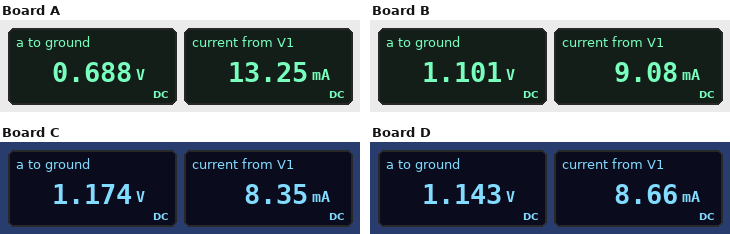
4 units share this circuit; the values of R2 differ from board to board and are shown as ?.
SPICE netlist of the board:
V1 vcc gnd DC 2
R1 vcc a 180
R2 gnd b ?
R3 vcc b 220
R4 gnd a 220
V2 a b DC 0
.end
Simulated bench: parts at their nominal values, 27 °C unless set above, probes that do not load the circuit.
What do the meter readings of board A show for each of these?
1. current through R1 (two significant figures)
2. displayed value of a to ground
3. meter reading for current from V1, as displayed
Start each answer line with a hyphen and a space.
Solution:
- 7.3 mA
- 0.688 V
- 13.25 mA
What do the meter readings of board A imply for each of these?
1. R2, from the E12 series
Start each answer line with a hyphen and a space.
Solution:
- 68 Ω
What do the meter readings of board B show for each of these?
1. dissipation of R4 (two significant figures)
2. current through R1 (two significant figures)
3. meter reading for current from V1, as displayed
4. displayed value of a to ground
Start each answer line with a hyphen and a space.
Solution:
- 5.5 mW
- 5.0 mA
- 9.08 mA
- 1.101 V
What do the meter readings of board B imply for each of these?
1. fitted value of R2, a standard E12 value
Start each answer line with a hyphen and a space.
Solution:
- 270 Ω
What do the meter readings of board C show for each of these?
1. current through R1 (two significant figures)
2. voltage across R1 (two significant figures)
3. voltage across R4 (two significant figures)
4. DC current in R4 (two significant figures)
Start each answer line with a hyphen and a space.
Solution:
- 4.6 mA
- 830 mV
- 1.2 V
- 5.3 mA
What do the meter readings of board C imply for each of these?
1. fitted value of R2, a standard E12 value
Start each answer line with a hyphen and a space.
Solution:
- 390 Ω
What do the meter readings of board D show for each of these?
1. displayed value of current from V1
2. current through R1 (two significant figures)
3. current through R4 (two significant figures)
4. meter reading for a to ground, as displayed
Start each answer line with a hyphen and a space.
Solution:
- 8.66 mA
- 4.8 mA
- 5.2 mA
- 1.143 V
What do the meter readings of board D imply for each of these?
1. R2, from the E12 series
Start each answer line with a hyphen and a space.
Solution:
- 330 Ω
